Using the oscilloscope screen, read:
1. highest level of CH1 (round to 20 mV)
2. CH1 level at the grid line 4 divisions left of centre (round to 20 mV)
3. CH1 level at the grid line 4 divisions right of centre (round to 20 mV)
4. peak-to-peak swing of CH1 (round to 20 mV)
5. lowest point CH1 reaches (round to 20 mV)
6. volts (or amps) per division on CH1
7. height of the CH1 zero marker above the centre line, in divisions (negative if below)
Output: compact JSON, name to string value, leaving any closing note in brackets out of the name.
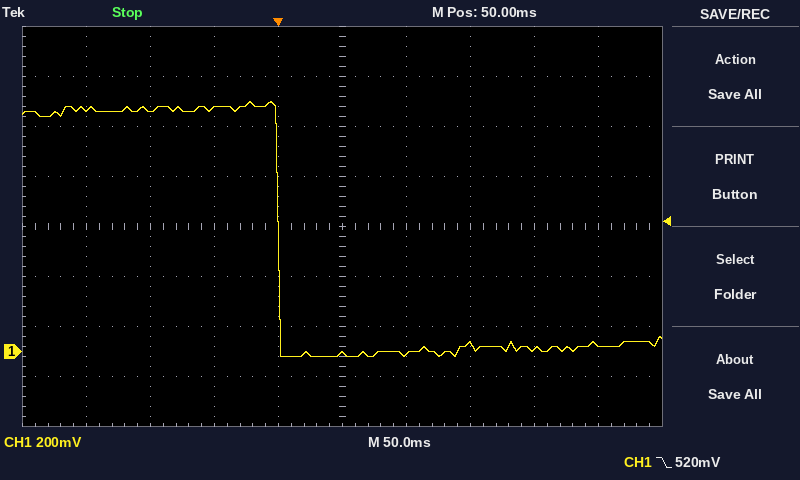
{"highest level of CH1": "1.00 V", "CH1 level at the grid line 4 divisions left of centre": "960 mV", "CH1 level at the grid line 4 divisions right of centre": "20 mV", "peak-to-peak swing of CH1": "1.02 V", "lowest point CH1 reaches": "-20 mV", "volts (or amps) per division on CH1": "200 mV", "height of the CH1 zero marker above the centre line, in divisions": "-2.5 div"}
